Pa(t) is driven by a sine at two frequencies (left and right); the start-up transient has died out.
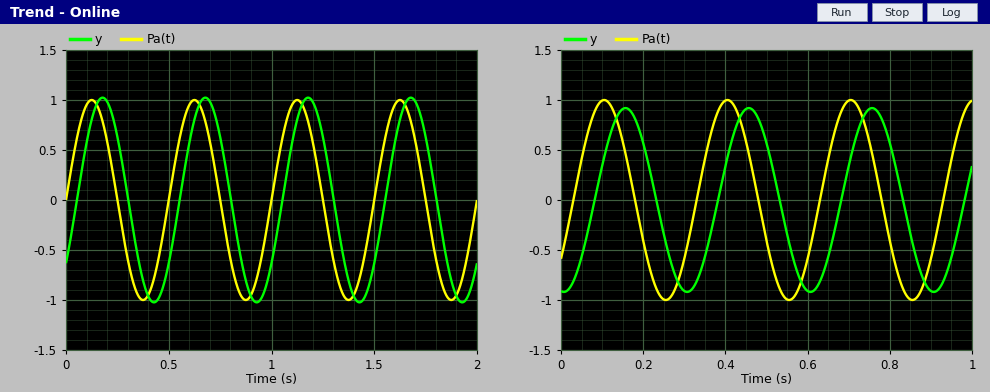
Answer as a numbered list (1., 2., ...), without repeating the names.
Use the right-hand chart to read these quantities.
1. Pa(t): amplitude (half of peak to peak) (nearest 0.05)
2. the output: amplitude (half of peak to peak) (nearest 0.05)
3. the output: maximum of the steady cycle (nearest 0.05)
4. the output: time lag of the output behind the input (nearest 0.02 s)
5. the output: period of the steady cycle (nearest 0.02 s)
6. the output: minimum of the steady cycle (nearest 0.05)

1. 1.00
2. 0.90
3. 0.90
4. 0.06 s
5. 0.30 s
6. -0.90
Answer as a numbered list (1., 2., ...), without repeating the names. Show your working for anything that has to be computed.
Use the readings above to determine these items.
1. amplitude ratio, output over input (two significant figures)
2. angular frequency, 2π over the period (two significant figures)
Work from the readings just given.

1. 0.9 / 1 = 0.90
2. 2π / 0.3 = 21 rad/s
